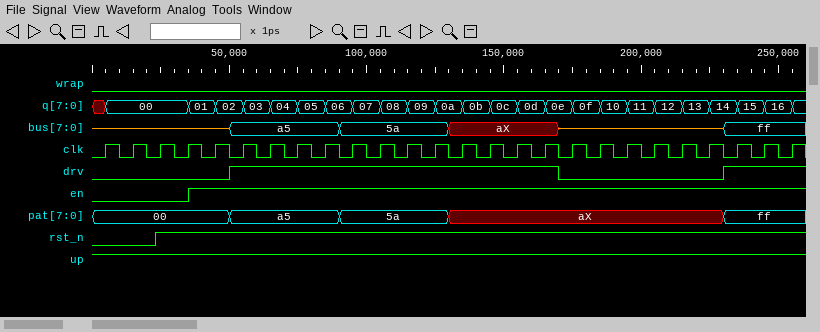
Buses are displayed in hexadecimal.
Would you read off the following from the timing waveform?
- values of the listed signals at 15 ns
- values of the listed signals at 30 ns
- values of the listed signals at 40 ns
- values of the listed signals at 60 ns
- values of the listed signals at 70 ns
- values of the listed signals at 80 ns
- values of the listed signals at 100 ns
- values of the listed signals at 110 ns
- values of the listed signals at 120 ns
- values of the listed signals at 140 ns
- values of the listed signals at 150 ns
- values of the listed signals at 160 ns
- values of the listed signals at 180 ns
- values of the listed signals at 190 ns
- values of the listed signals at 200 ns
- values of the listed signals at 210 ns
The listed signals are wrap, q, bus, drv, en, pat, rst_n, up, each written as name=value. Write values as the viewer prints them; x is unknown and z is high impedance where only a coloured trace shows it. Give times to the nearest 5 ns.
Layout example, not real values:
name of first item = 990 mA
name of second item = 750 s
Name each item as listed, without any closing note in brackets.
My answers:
values of the listed signals at 15 ns = wrap=0, q=00, bus=z, drv=0, en=0, pat=00, rst_n=0, up=1
values of the listed signals at 30 ns = wrap=0, q=00, bus=z, drv=0, en=0, pat=00, rst_n=1, up=1
values of the listed signals at 40 ns = wrap=0, q=01, bus=z, drv=0, en=1, pat=00, rst_n=1, up=1
values of the listed signals at 60 ns = wrap=0, q=03, bus=a5, drv=1, en=1, pat=a5, rst_n=1, up=1
values of the listed signals at 70 ns = wrap=0, q=04, bus=a5, drv=1, en=1, pat=a5, rst_n=1, up=1
values of the listed signals at 80 ns = wrap=0, q=05, bus=a5, drv=1, en=1, pat=a5, rst_n=1, up=1
values of the listed signals at 100 ns = wrap=0, q=07, bus=5a, drv=1, en=1, pat=5a, rst_n=1, up=1
values of the listed signals at 110 ns = wrap=0, q=08, bus=5a, drv=1, en=1, pat=5a, rst_n=1, up=1
values of the listed signals at 120 ns = wrap=0, q=09, bus=5a, drv=1, en=1, pat=5a, rst_n=1, up=1
values of the listed signals at 140 ns = wrap=0, q=0b, bus=aX, drv=1, en=1, pat=aX, rst_n=1, up=1
values of the listed signals at 150 ns = wrap=0, q=0c, bus=aX, drv=1, en=1, pat=aX, rst_n=1, up=1
values of the listed signals at 160 ns = wrap=0, q=0d, bus=aX, drv=1, en=1, pat=aX, rst_n=1, up=1
values of the listed signals at 180 ns = wrap=0, q=0f, bus=z, drv=0, en=1, pat=aX, rst_n=1, up=1
values of the listed signals at 190 ns = wrap=0, q=10, bus=z, drv=0, en=1, pat=aX, rst_n=1, up=1
values of the listed signals at 200 ns = wrap=0, q=11, bus=z, drv=0, en=1, pat=aX, rst_n=1, up=1
values of the listed signals at 210 ns = wrap=0, q=12, bus=z, drv=0, en=1, pat=aX, rst_n=1, up=1
